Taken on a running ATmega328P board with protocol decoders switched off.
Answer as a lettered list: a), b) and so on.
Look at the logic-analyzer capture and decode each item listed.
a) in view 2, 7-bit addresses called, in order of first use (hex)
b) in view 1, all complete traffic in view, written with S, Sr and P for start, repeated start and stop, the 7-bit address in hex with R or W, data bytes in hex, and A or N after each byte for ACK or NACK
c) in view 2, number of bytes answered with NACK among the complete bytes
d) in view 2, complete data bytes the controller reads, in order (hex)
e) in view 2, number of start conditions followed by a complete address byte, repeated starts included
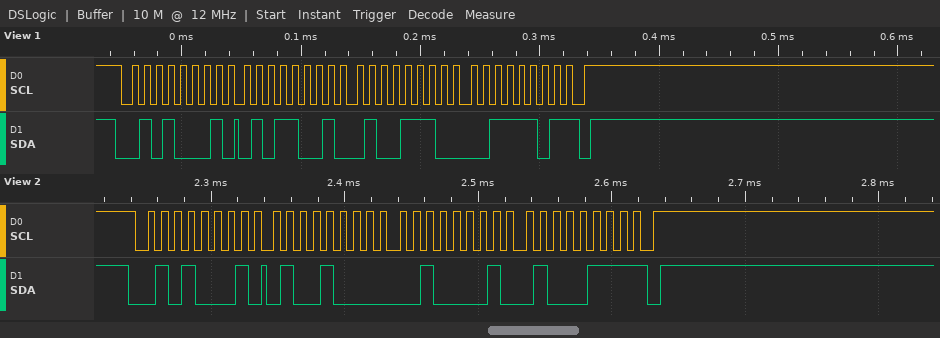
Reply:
a) 0x28
b) S 28R A 59 A 4E A 3D N P
c) 1
d) 48 21 47
e) 1
